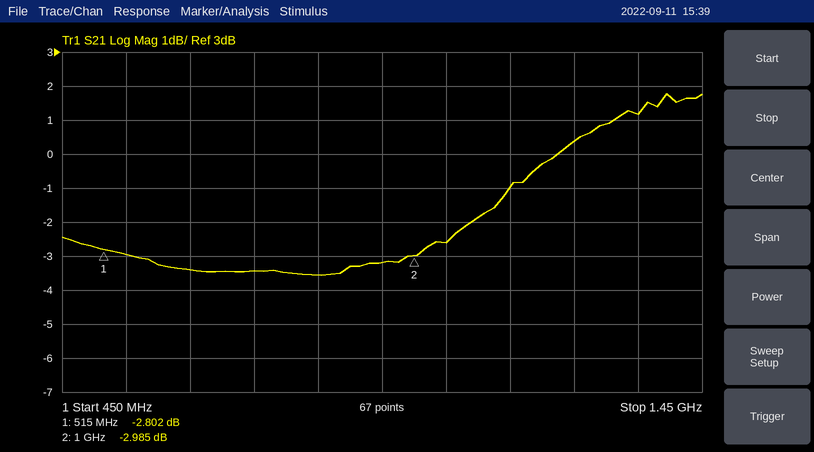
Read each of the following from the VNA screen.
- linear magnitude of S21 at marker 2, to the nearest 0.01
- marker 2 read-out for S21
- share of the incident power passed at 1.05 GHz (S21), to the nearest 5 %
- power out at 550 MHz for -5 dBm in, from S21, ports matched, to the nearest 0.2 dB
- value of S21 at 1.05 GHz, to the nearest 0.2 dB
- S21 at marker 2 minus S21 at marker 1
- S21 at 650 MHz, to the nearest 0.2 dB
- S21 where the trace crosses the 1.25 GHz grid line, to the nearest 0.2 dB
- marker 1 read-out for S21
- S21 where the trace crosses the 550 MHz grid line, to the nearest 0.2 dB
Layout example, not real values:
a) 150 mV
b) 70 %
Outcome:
a) 0.71
b) -2.985 dB
c) 55 %
d) -8.0 dBm
e) -2.6 dB
f) -0.183 dB
g) -3.4 dB
h) 0.4 dB
i) -2.802 dB
j) -3.0 dB
